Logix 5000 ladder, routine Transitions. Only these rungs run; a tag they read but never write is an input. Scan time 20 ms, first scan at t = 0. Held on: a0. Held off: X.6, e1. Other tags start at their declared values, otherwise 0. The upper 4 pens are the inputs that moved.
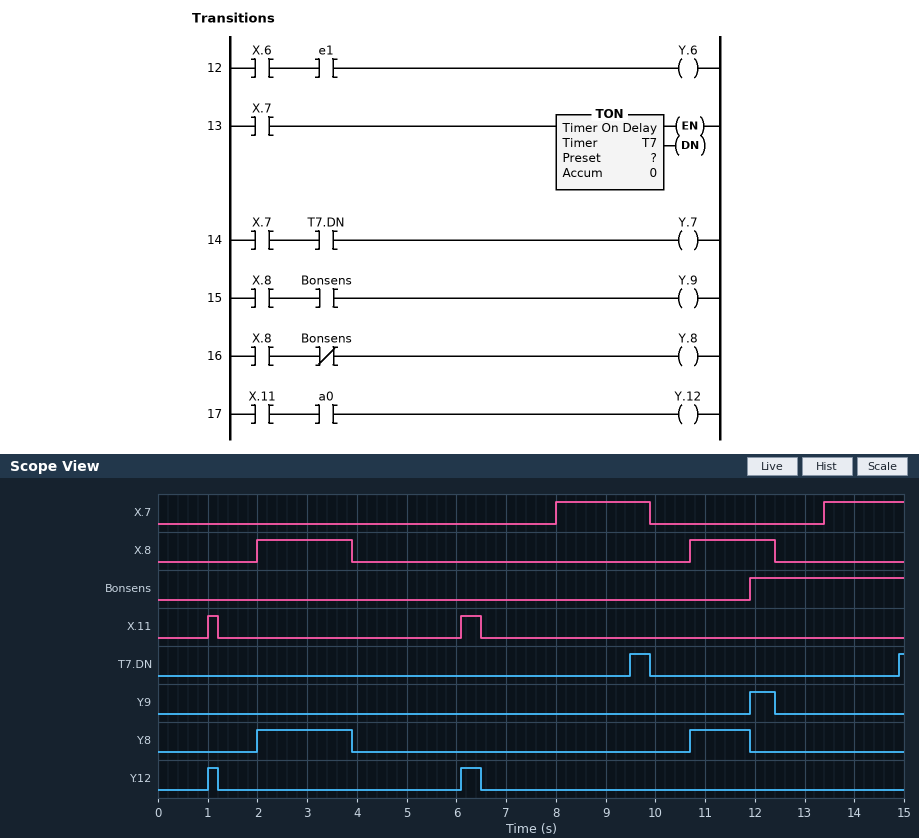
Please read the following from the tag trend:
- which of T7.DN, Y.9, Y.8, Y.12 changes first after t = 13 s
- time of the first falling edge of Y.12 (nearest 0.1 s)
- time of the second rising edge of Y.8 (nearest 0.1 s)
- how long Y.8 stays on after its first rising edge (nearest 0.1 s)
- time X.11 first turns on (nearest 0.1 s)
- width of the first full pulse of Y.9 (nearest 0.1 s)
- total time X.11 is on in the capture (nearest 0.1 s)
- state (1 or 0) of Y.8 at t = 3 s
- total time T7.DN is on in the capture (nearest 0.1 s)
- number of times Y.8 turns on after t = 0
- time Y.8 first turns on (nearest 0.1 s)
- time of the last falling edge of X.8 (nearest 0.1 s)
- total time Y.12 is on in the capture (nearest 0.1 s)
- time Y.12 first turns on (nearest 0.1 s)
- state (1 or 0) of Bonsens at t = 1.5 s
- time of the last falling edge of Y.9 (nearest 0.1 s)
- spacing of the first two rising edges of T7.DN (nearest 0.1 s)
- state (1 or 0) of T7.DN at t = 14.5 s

T7.DN
1.2 s
10.7 s
1.9 s
1.0 s
0.5 s
0.6 s
1
0.5 s
2
2.0 s
12.4 s
0.6 s
1.0 s
0
12.4 s
5.4 s
0
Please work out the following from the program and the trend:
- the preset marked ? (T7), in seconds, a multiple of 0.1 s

1.5 s
